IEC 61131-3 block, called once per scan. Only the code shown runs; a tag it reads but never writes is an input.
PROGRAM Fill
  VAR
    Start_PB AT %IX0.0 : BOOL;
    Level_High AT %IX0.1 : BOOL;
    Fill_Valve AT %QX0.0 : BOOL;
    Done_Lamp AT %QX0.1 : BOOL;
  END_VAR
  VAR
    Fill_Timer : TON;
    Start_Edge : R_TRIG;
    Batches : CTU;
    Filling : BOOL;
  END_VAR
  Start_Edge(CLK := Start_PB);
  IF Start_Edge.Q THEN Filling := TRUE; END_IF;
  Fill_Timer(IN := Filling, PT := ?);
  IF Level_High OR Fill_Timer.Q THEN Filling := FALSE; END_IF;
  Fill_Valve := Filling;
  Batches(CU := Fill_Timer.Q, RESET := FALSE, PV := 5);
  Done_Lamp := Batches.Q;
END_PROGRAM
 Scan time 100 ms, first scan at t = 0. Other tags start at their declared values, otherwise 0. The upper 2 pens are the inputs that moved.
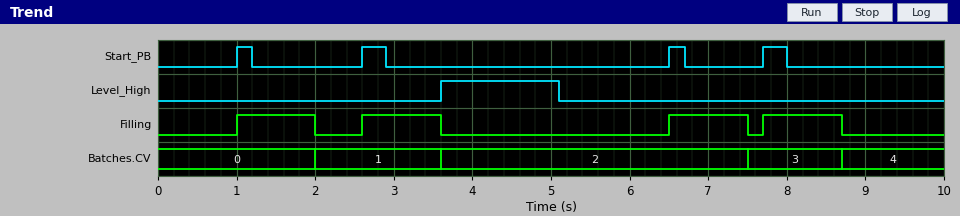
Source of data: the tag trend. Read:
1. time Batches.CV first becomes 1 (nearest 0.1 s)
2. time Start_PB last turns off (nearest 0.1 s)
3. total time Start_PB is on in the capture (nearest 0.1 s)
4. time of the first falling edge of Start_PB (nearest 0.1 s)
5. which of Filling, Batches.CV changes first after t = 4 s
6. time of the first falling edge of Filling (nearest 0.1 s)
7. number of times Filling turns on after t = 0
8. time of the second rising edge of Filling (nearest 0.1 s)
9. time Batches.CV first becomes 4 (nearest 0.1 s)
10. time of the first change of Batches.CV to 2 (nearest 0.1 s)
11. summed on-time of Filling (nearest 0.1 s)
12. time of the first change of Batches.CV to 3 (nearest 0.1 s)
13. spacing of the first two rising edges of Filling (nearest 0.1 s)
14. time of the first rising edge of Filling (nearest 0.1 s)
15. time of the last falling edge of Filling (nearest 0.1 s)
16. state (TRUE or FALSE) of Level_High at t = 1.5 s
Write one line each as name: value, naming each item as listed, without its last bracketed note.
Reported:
time Batches.CV first becomes 1: 2.0 s
time Start_PB last turns off: 8.0 s
total time Start_PB is on in the capture: 1.0 s
time of the first falling edge of Start_PB: 1.2 s
which of Filling, Batches.CV changes first after t = 4 s: Filling
time of the first falling edge of Filling: 2.0 s
number of times Filling turns on after t = 0: 4
time of the second rising edge of Filling: 2.6 s
time Batches.CV first becomes 4: 8.7 s
time of the first change of Batches.CV to 2: 3.6 s
summed on-time of Filling: 4.0 s
time of the first change of Batches.CV to 3: 7.5 s
spacing of the first two rising edges of Filling: 1.6 s
time of the first rising edge of Filling: 1.0 s
time of the last falling edge of Filling: 8.7 s
state (TRUE or FALSE) of Level_High at t = 1.5 s: FALSE
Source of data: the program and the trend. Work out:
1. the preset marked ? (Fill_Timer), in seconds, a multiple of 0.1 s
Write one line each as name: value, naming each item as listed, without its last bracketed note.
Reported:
the preset marked ? (Fill_Timer), in seconds, a multiple of 0.1 s: 1.0 s
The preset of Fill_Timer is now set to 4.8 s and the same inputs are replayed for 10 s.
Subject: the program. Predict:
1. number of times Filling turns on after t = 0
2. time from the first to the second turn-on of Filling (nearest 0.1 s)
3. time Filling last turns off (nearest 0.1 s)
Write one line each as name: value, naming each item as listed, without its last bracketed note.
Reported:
number of times Filling turns on after t = 0: 2
time from the first to the second turn-on of Filling: 5.5 s
time Filling last turns off: 3.6 s
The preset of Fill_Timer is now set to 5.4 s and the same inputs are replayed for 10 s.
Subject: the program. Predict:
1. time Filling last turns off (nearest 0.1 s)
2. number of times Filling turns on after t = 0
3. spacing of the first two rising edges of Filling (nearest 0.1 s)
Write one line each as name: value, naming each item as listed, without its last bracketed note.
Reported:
time Filling last turns off: 3.6 s
number of times Filling turns on after t = 0: 2
spacing of the first two rising edges of Filling: 5.5 s
